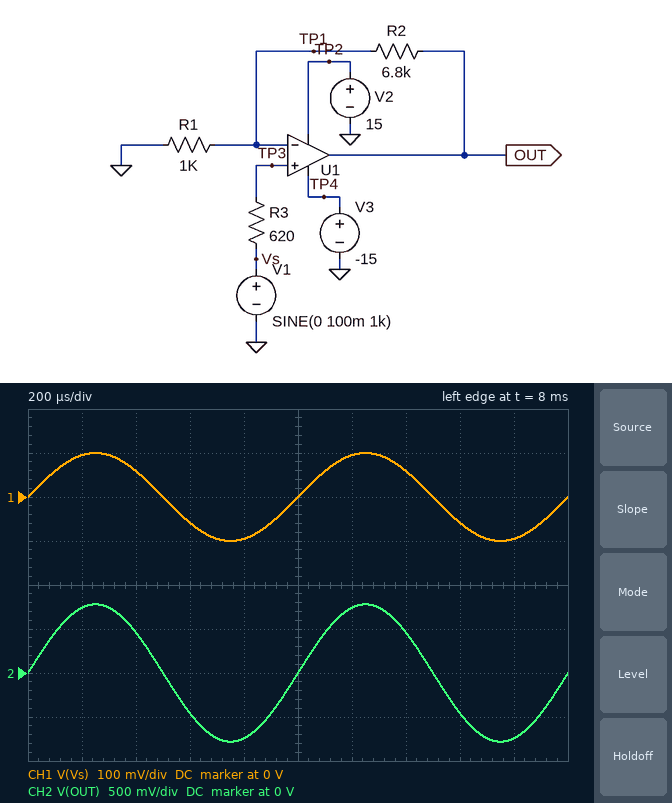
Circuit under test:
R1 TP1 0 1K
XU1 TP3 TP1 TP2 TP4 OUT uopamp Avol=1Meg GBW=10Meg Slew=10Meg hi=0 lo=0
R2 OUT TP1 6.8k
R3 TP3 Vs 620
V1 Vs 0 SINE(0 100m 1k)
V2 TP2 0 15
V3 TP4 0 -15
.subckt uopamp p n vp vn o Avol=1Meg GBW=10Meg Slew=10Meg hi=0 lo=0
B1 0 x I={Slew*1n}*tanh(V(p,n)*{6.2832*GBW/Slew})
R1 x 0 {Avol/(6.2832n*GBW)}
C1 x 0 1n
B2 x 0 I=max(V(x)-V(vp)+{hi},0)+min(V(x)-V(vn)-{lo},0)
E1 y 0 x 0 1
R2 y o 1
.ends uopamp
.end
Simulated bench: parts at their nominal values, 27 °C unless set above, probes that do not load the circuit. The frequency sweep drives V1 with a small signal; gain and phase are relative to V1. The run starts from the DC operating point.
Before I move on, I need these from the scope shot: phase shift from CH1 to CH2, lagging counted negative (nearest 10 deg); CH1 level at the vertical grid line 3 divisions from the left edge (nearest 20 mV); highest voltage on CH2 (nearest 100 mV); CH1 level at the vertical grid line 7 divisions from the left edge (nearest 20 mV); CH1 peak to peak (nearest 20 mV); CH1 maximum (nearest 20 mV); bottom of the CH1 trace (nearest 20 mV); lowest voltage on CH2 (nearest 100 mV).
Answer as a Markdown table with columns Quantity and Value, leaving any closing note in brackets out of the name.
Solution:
| Quantity | Value |
|---|---|
| phase shift from CH1 to CH2, lagging counted negative | 0 deg |
| CH1 level at the vertical grid line 3 divisions from the left edge | -60 mV |
| highest voltage on CH2 | 800 mV |
| CH1 level at the vertical grid line 7 divisions from the left edge | 60 mV |
| CH1 peak to peak | 200 mV |
| CH1 maximum | 100 mV |
| bottom of the CH1 trace | -100 mV |
| lowest voltage on CH2 | -800 mV |
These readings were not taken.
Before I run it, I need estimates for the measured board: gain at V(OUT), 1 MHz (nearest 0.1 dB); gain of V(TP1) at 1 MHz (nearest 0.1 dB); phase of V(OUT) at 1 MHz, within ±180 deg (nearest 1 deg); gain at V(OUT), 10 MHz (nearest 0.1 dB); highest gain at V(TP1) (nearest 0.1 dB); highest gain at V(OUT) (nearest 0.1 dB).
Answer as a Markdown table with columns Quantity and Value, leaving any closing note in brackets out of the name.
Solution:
| Quantity | Value |
|---|---|
| gain at V(OUT), 1 MHz | 15.8 dB |
| gain of V(TP1) at 1 MHz | -2.1 dB |
| phase of V(OUT) at 1 MHz, within ±180 deg | -38 deg |
| gain at V(OUT), 10 MHz | -0.1 dB |
| highest gain at V(TP1) | 0 dB |
| highest gain at V(OUT) | 17.8 dB |
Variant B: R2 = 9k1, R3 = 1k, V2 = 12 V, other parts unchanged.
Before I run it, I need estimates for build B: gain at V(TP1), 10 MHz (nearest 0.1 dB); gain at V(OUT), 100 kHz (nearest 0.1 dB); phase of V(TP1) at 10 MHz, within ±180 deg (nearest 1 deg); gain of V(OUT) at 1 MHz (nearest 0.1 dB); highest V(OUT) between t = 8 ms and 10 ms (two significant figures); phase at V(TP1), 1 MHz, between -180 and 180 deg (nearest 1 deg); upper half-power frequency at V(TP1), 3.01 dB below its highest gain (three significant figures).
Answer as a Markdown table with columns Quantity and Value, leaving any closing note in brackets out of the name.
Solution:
| Quantity | Value |
|---|---|
| gain at V(TP1), 10 MHz | -20.1 dB |
| gain at V(OUT), 100 kHz | 20.0 dB |
| phase of V(TP1) at 10 MHz, within ±180 deg | -84 deg |
| gain of V(OUT) at 1 MHz | 17.0 dB |
| highest V(OUT) between t = 8 ms and 10 ms | 1.0 V |
| phase at V(TP1), 1 MHz, between -180 and 180 deg | -45 deg |
| upper half-power frequency at V(TP1), 3.01 dB below its highest gain | 990 kHz |
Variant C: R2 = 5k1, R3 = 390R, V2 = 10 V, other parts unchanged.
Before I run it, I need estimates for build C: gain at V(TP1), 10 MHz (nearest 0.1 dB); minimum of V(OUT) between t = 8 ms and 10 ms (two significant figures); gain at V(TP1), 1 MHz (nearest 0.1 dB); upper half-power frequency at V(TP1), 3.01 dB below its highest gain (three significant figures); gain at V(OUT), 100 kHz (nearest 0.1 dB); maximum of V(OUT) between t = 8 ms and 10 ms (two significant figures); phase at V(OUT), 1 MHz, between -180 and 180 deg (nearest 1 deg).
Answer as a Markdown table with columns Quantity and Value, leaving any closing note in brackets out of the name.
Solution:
| Quantity | Value |
|---|---|
| gain at V(TP1), 10 MHz | -15.8 dB |
| minimum of V(OUT) between t = 8 ms and 10 ms | -610 mV |
| gain at V(TP1), 1 MHz | -1.4 dB |
| upper half-power frequency at V(TP1), 3.01 dB below its highest gain | 1.64 MHz |
| gain at V(OUT), 100 kHz | 15.7 dB |
| maximum of V(OUT) between t = 8 ms and 10 ms | 610 mV |
| phase at V(OUT), 1 MHz, between -180 and 180 deg | -31 deg |
